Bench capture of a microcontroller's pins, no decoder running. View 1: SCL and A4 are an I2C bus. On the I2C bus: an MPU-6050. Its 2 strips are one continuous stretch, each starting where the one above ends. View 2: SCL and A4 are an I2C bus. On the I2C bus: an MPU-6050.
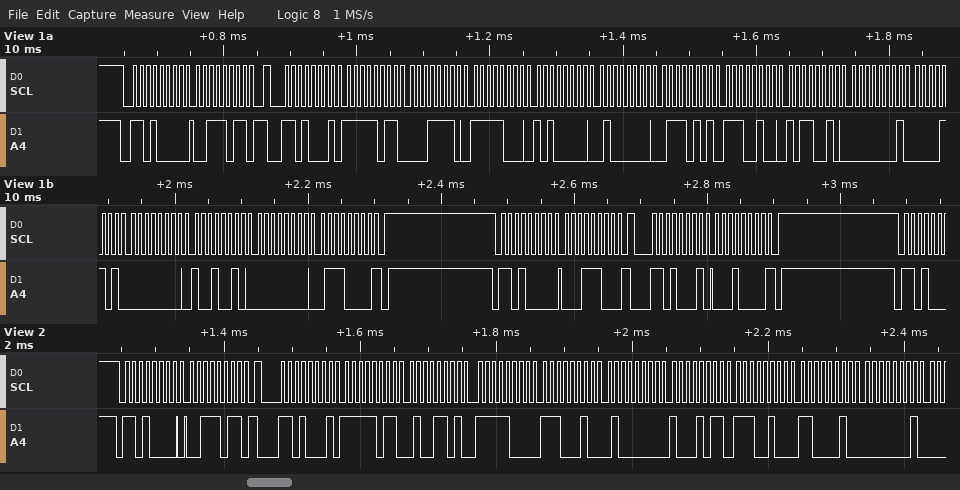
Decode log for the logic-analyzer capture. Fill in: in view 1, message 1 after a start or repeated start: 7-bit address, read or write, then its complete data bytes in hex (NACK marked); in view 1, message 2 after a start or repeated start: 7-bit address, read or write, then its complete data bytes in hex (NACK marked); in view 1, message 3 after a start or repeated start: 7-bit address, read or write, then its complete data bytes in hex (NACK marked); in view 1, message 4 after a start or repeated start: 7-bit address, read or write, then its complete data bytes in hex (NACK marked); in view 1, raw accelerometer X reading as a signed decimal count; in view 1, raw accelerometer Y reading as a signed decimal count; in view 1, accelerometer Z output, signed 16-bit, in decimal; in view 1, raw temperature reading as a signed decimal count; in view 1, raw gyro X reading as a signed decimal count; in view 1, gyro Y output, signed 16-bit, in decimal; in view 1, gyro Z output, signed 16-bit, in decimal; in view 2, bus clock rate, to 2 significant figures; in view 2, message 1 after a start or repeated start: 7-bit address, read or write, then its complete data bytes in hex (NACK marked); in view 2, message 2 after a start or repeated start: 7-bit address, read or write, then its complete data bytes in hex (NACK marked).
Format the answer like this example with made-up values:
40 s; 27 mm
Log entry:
0x68 write: 3B; 0x68 read: FB 1E F8 A0 40 75 E4 B2 01 0D 00 92 00 70 NACK; 0x68 write: 1C; 0x68 read: 10 NACK; -1250; -1888; 16501; -6990; 269; 146; 112; 100 kHz; 0x68 write: 3B; 0x68 read: FB 4D F8 E2 40 8B E4 C2 01
